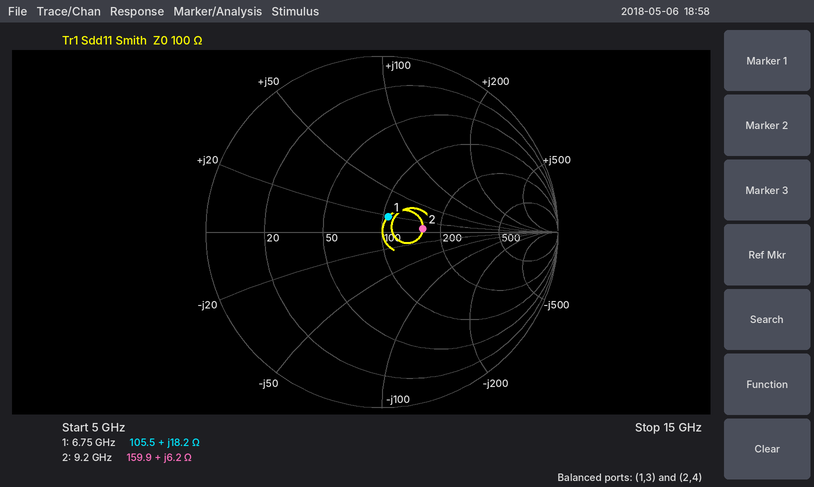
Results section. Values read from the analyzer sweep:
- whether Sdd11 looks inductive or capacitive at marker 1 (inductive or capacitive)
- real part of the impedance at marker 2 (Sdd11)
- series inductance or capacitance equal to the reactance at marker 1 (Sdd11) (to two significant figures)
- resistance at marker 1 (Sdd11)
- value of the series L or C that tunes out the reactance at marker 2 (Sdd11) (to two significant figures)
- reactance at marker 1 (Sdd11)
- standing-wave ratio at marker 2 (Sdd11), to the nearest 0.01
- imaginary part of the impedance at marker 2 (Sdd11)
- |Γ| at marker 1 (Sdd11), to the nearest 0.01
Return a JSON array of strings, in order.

["inductive", "159.9 Ω", "430 pH", "105.5 Ω", "2.8 pF", "+18.2 Ω", "1.60", "+6.2 Ω", "0.09"]
